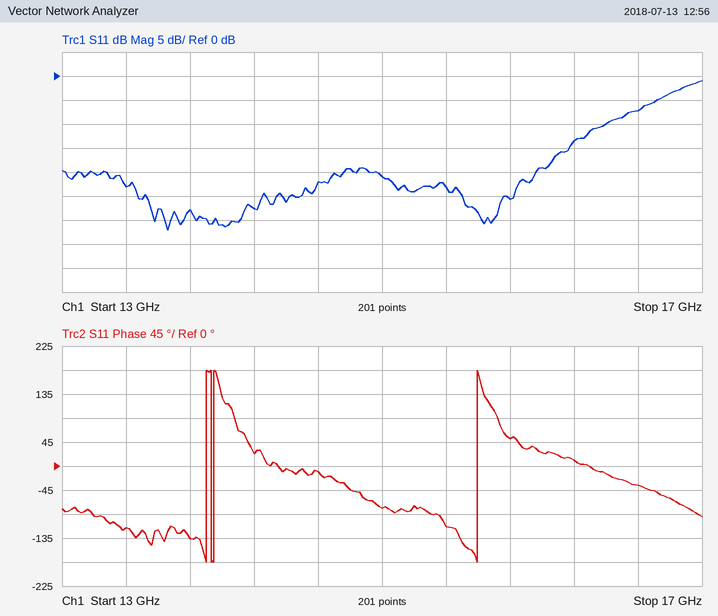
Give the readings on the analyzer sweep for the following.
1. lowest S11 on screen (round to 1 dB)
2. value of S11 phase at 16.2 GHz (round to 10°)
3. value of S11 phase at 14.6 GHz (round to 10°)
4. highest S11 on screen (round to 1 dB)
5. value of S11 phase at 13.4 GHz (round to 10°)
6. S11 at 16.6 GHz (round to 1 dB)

-32 dB
10°
-10°
-1 dB
-120°
-7 dB
